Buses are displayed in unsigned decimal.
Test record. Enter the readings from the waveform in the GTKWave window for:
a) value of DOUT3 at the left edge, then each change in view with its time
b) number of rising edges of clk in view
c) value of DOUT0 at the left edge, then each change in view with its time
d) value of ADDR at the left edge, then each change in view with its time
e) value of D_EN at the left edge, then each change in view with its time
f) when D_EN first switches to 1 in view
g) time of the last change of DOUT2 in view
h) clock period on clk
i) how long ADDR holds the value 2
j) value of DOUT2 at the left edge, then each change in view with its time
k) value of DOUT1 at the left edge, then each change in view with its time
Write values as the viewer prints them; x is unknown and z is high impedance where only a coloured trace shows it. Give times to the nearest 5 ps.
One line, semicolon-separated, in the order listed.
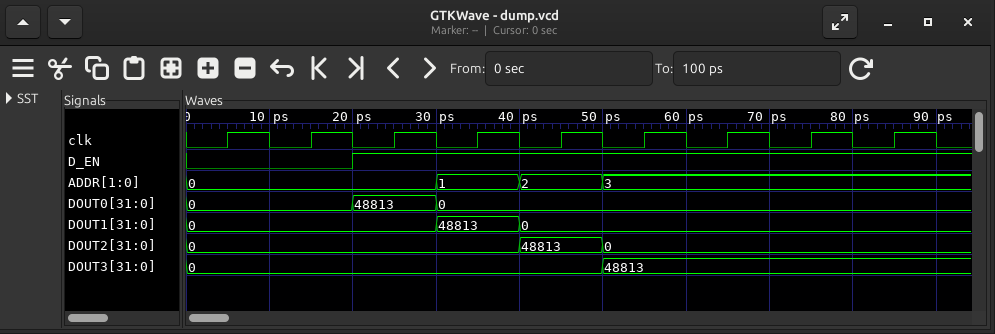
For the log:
0, 48813 at 50 ps; 9; 0, 48813 at 20 ps, 0 at 30 ps; 0, 1 at 30 ps, 2 at 40 ps, 3 at 50 ps; 0, 1 at 20 ps; 20 ps; 50 ps; 10 ps; 10 ps; 0, 48813 at 40 ps, 0 at 50 ps; 0, 48813 at 30 ps, 0 at 40 ps
